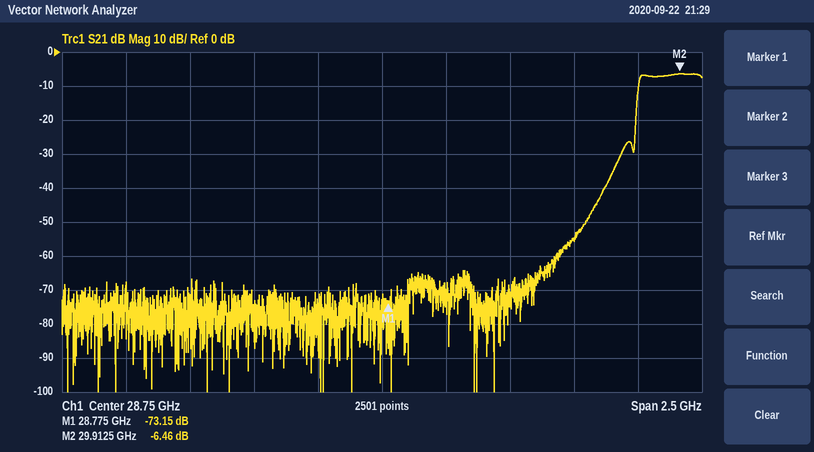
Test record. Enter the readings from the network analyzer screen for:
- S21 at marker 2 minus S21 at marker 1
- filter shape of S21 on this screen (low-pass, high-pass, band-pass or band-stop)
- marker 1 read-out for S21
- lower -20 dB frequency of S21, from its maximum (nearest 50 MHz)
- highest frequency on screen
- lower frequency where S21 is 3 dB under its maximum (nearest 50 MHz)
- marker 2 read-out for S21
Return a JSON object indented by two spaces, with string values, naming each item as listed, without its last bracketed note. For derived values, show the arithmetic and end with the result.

{
  "S21 at marker 2 minus S21 at marker 1": "-6.46 − (-73.15) = 66.69 dB",
  "filter shape of S21 on this screen": "high-pass",
  "marker 1 read-out for S21": "-73.15 dB",
  "lower -20 dB frequency of S21, from its maximum": "29.75 GHz",
  "highest frequency on screen": "30 GHz",
  "lower frequency where S21 is 3 dB under its maximum": "29.75 GHz",
  "marker 2 read-out for S21": "-6.46 dB"
}
